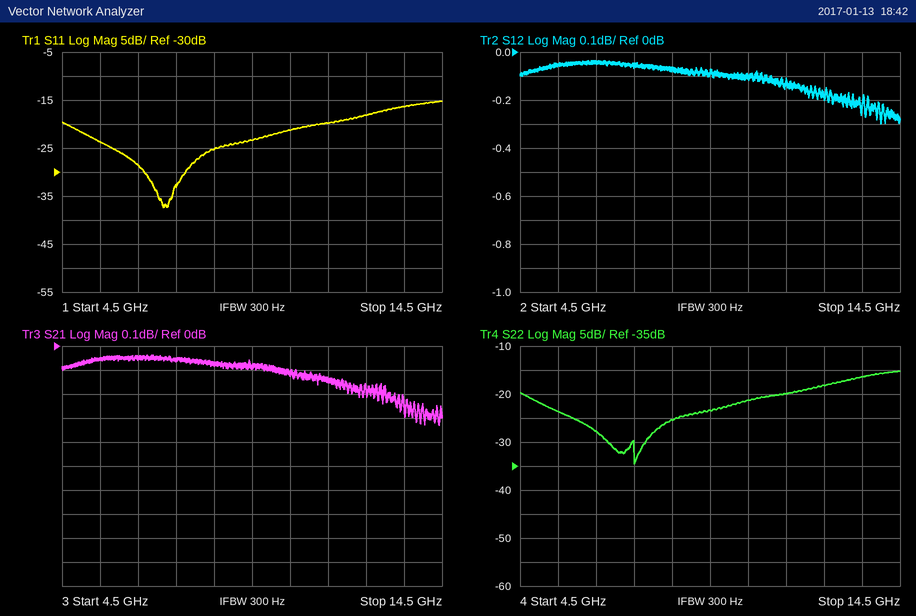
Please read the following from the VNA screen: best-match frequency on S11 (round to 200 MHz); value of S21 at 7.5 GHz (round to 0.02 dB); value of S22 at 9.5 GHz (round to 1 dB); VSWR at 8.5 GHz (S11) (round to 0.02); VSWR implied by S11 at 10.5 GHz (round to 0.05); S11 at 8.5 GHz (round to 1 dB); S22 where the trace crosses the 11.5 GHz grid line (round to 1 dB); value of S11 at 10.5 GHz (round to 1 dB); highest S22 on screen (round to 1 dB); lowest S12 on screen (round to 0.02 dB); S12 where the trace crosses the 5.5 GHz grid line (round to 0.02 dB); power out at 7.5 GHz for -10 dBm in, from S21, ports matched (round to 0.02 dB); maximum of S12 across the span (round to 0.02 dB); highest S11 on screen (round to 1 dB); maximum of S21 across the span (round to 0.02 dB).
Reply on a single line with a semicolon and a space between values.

7.2 GHz; -0.06 dB; -23 dB; 1.12; 1.20; -25 dB; -20 dB; -21 dB; -15 dB; -0.30 dB; -0.06 dB; -10.06 dBm; -0.04 dB; -15 dB; -0.04 dB
